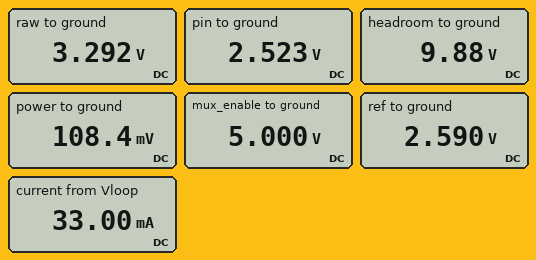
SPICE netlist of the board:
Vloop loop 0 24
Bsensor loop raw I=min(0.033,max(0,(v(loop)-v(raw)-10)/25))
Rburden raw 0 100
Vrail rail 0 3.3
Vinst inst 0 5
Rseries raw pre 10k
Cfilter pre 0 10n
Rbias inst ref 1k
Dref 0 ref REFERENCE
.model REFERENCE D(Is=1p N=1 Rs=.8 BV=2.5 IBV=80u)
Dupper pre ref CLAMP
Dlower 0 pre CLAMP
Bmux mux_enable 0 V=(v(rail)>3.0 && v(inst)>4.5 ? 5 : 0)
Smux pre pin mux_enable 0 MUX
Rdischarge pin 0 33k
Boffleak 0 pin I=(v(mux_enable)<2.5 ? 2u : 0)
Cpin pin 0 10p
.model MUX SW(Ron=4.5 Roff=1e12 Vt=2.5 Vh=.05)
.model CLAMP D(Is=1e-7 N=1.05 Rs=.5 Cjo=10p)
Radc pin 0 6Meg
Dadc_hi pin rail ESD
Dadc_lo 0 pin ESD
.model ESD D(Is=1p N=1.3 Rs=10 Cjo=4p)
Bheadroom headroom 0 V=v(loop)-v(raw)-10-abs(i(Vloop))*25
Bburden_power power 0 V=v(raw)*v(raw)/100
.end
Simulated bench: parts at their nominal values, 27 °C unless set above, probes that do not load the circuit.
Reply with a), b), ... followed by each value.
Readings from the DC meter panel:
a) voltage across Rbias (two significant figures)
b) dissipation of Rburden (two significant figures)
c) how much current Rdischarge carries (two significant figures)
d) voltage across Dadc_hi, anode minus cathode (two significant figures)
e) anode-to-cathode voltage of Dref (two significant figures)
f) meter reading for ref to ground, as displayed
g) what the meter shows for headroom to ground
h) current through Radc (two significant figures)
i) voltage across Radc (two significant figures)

a) 2.4 V
b) 110 mW
c) 76 µA
d) -780 mV
e) -2.6 V
f) 2.590 V
g) 9.88 V
h) 420 nA
i) 2.5 V
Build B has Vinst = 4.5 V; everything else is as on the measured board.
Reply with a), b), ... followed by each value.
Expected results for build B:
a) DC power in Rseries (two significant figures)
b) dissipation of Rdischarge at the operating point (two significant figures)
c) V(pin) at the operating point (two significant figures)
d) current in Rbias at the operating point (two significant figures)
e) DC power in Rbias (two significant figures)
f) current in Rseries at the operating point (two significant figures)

a) 29 µW
b) 130 nW
c) 66 mV
d) 1.9 mA
e) 3.7 mW
f) 54 µA
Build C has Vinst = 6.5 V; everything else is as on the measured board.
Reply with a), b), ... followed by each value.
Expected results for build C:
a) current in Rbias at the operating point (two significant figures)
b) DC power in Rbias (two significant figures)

a) 3.9 mA
b) 15 mW
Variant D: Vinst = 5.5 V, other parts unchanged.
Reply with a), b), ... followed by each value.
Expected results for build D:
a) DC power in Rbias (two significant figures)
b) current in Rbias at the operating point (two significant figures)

a) 8.4 mW
b) 2.9 mA
